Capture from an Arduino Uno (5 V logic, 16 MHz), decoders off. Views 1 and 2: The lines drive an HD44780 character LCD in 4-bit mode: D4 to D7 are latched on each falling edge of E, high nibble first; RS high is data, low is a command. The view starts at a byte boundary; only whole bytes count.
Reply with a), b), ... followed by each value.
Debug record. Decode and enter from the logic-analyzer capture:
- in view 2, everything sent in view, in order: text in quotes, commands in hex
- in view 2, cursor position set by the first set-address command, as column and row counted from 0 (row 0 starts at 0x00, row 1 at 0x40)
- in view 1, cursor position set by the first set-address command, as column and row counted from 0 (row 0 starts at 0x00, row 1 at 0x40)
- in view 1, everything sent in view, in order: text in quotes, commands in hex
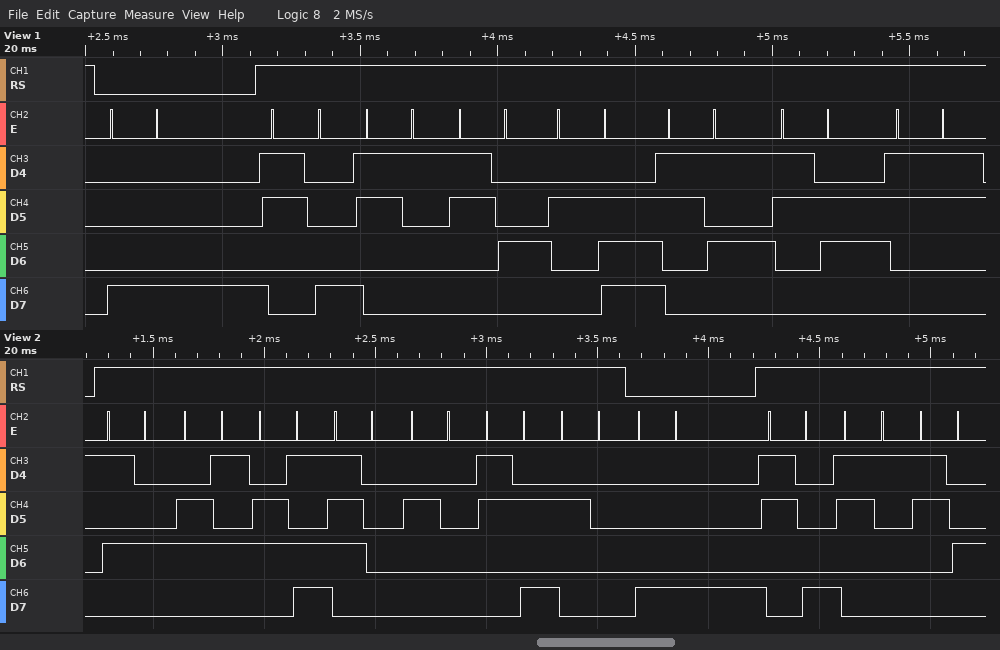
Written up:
a) "Temp : " 0x88 "814"
b) column 8, row 0
c) column 8, row 0
d) 0x88 "814.563"
